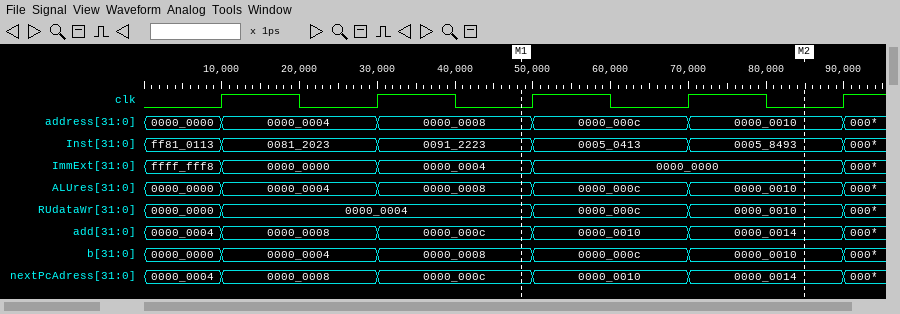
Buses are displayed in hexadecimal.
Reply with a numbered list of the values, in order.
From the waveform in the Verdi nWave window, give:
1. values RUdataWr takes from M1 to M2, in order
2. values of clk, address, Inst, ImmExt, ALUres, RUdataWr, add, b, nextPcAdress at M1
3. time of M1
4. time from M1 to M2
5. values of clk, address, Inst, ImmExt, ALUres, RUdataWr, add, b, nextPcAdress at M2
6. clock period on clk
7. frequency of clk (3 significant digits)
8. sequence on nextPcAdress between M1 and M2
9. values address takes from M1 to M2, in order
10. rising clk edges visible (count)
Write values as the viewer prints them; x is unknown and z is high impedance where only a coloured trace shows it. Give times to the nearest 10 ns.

1. 0000_0004, 0000_000c, 0000_0010
2. clk=0, address=0000_0008, Inst=0091_2223, ImmExt=0000_0004, ALUres=0000_0008, RUdataWr=0000_0004, add=0000_000c, b=0000_0008, nextPcAdress=0000_000c
3. 50 ns
4. 40 ns
5. clk=0, address=0000_0010, Inst=0005_8493, ImmExt=0000_0000, ALUres=0000_0010, RUdataWr=0000_0010, add=0000_0014, b=0000_0010, nextPcAdress=0000_0014
6. 20 ns
7. 50.0 MHz
8. 0000_000c, 0000_0010, 0000_0014
9. 0000_0008, 0000_000c, 0000_0010
10. 5
